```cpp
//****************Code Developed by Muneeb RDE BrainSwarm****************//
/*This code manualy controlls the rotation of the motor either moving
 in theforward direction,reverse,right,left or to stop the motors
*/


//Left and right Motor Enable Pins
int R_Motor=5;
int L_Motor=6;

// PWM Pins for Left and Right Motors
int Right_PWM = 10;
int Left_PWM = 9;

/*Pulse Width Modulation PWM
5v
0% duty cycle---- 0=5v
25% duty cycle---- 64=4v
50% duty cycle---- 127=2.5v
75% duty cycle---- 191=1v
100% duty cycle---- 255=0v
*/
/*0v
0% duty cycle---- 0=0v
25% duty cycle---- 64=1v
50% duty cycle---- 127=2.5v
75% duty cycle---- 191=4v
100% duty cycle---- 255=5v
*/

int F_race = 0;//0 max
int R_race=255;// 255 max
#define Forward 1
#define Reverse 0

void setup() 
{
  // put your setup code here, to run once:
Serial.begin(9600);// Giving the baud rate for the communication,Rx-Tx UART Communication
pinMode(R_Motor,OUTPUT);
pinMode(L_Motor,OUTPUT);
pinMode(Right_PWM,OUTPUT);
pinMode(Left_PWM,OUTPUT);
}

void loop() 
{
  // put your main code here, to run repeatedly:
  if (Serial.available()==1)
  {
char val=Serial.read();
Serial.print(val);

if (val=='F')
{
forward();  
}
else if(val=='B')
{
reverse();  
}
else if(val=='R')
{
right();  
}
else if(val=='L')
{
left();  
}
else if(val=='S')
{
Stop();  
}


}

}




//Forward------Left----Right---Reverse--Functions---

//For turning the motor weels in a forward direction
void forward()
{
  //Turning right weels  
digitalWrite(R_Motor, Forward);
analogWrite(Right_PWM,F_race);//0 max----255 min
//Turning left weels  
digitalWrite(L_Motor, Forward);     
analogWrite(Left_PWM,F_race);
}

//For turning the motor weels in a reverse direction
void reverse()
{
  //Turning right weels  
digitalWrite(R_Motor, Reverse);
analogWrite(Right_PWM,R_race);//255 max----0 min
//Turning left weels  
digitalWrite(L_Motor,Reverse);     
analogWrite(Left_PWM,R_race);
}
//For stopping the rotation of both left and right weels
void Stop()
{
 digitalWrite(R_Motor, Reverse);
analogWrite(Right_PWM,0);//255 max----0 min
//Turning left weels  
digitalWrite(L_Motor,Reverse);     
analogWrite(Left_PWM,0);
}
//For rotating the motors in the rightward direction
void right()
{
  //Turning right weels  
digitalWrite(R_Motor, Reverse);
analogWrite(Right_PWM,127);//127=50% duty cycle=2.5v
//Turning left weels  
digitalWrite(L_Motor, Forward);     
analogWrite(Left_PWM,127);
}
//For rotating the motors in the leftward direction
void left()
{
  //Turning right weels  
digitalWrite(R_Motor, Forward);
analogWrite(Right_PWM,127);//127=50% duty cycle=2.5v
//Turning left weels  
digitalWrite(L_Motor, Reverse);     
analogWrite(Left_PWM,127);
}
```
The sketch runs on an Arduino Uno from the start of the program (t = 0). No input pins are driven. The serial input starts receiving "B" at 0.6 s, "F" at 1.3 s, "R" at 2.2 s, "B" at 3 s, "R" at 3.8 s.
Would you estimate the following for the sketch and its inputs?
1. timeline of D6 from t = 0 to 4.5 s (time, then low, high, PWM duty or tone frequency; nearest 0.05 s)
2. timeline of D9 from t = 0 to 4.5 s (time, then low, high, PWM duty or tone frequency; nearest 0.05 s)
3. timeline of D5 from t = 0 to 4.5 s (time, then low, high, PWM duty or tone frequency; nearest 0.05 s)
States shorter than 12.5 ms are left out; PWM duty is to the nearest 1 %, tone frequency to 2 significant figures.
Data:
0 s low; 1.3 s high; 3 s low; 3.8 s high
0 s low; 0.6 s high; 1.3 s low; 2.2 s PWM 50 %; 3 s high; 3.8 s PWM 50 %
0 s low; 1.3 s high; 2.2 s low
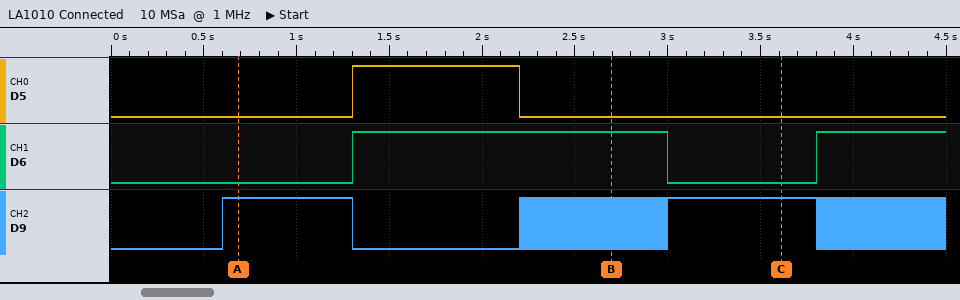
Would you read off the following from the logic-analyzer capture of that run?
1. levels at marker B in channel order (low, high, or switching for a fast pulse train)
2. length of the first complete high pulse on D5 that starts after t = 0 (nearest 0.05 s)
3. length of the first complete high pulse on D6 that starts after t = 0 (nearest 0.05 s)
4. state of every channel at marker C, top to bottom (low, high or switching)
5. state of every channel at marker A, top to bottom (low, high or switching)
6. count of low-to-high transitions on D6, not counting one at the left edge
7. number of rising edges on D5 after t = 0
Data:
D5 low, D6 high, D9 switching
0.90 s
1.70 s
D5 low, D6 low, D9 high
D5 low, D6 low, D9 high
2
1
